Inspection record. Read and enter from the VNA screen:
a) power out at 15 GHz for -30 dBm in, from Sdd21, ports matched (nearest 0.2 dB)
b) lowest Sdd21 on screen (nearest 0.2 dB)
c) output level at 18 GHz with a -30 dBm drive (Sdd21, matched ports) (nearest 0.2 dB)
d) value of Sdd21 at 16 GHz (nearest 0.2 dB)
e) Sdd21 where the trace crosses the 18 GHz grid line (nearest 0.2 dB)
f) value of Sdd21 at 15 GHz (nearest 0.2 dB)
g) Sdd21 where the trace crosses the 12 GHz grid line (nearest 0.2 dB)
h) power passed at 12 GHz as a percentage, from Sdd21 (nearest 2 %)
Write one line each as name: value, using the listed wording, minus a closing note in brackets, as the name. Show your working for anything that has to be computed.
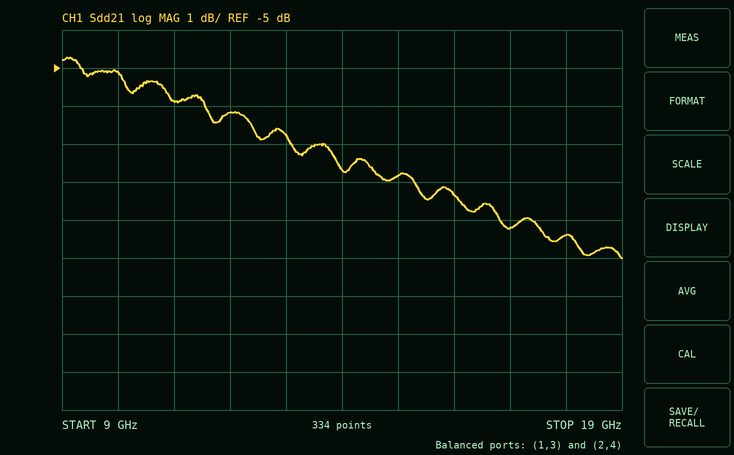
power out at 15 GHz for -30 dBm in, from Sdd21, ports matched: -30 dBm + (-7.8 dB) = -37.8 dBm
lowest Sdd21 on screen: -10.0 dB
output level at 18 GHz with a -30 dBm drive (Sdd21, matched ports): -30 dBm + (-9.4 dB) = -39.4 dBm
value of Sdd21 at 16 GHz: -8.4 dB
Sdd21 where the trace crosses the 18 GHz grid line: -9.4 dB
value of Sdd21 at 15 GHz: -7.8 dB
Sdd21 where the trace crosses the 12 GHz grid line: -6.2 dB
power passed at 12 GHz as a percentage, from Sdd21: 10^(-6.2/10) ≈ 24 %
